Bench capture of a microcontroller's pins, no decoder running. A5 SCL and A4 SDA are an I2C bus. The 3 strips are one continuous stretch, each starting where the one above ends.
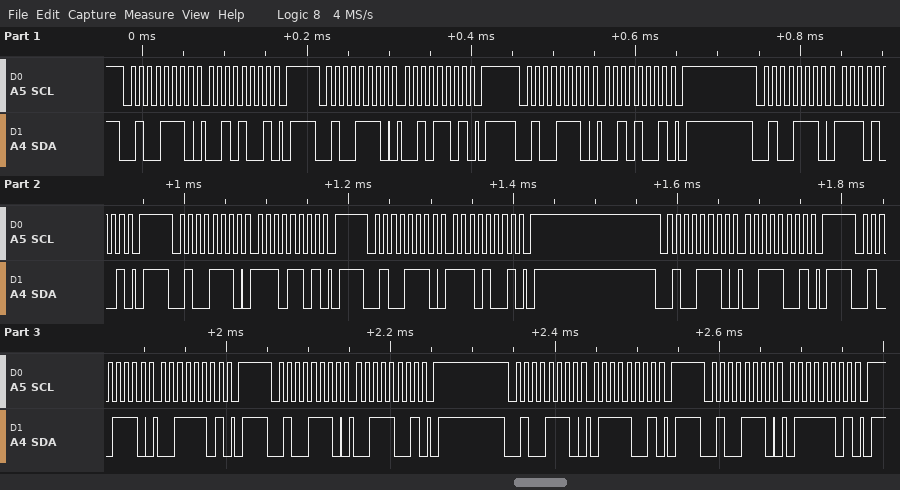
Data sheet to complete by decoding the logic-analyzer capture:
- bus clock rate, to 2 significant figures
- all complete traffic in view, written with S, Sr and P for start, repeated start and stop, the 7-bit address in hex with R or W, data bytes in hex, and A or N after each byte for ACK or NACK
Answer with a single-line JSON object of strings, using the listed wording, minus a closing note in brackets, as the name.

{"bus clock rate, to 2 significant figures": "100 kHz", "all complete traffic in view, written with S, Sr and P for start, repeated start and stop, the 7-bit address in hex with R or W, data bytes in hex, and A or N after each byte for ACK or NACK": "S 27W A 29 A P S 27W A 2D A P S 27W A 29 A P S 27W A E9 A P S 27W A ED A P S 27W A E9 A P S 27W A 39 A P S 27W A 3D A P S 27W A 39 A P S 27W A 79 A P S 27W A 7D A P"}
